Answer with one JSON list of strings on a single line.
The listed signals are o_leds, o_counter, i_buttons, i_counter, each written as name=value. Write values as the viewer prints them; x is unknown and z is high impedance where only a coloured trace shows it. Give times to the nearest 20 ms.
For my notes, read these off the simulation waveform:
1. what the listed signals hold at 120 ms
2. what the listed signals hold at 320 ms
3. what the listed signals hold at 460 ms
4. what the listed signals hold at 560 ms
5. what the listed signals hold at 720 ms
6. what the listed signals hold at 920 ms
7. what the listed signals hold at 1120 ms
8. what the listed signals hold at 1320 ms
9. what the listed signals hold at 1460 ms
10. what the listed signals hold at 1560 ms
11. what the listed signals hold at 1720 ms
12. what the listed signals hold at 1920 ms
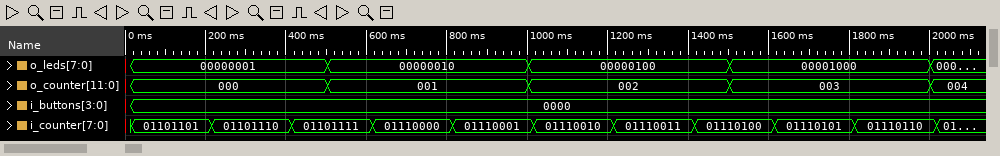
["o_leds=00000001, o_counter=000, i_buttons=0000, i_counter=01101101", "o_leds=00000001, o_counter=000, i_buttons=0000, i_counter=01101110", "o_leds=00000001, o_counter=000, i_buttons=0000, i_counter=01101111", "o_leds=00000010, o_counter=001, i_buttons=0000, i_counter=01101111", "o_leds=00000010, o_counter=001, i_buttons=0000, i_counter=01110000", "o_leds=00000010, o_counter=001, i_buttons=0000, i_counter=01110001", "o_leds=00000100, o_counter=002, i_buttons=0000, i_counter=01110010", "o_leds=00000100, o_counter=002, i_buttons=0000, i_counter=01110011", "o_leds=00000100, o_counter=002, i_buttons=0000, i_counter=01110100", "o_leds=00001000, o_counter=003, i_buttons=0000, i_counter=01110100", "o_leds=00001000, o_counter=003, i_buttons=0000, i_counter=01110101", "o_leds=00001000, o_counter=003, i_buttons=0000, i_counter=01110110"]
